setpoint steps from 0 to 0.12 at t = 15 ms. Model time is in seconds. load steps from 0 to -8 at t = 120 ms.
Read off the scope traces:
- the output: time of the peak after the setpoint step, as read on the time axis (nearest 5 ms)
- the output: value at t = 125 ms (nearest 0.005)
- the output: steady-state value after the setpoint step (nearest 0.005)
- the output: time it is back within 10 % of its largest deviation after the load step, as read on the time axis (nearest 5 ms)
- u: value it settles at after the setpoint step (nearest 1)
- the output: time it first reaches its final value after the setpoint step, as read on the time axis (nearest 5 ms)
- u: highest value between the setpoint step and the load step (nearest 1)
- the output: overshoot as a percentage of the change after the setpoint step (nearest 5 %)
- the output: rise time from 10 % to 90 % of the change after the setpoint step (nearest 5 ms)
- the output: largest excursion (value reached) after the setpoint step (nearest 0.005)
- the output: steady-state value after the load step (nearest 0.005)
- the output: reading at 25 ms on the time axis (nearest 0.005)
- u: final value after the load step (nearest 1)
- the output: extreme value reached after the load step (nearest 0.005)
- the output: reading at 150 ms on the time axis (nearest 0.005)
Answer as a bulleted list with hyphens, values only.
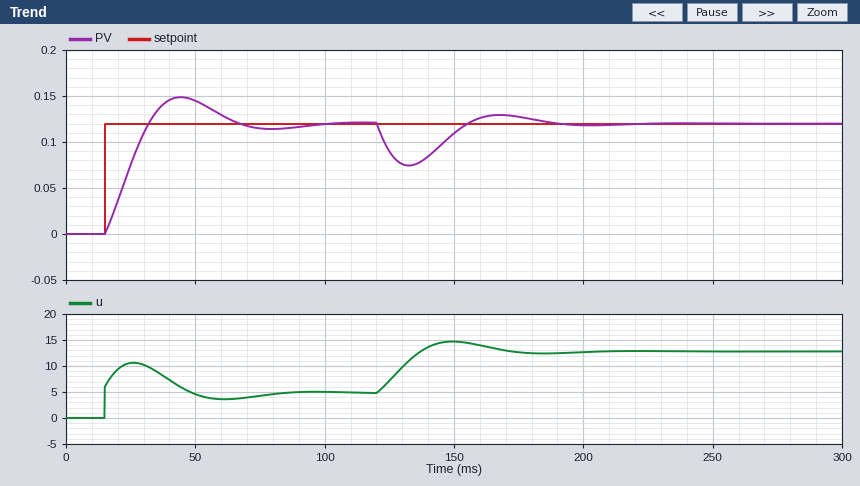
- 45 ms
- 0.090
- 0.120
- 180 ms
- 5
- 30 ms
- 11
- 25 %
- 15 ms
- 0.150
- 0.120
- 0.075
- 13
- 0.075
- 0.110
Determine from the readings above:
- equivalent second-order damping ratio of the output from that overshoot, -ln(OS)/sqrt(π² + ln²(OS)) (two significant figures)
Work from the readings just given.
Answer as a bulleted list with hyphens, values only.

- 0.40
